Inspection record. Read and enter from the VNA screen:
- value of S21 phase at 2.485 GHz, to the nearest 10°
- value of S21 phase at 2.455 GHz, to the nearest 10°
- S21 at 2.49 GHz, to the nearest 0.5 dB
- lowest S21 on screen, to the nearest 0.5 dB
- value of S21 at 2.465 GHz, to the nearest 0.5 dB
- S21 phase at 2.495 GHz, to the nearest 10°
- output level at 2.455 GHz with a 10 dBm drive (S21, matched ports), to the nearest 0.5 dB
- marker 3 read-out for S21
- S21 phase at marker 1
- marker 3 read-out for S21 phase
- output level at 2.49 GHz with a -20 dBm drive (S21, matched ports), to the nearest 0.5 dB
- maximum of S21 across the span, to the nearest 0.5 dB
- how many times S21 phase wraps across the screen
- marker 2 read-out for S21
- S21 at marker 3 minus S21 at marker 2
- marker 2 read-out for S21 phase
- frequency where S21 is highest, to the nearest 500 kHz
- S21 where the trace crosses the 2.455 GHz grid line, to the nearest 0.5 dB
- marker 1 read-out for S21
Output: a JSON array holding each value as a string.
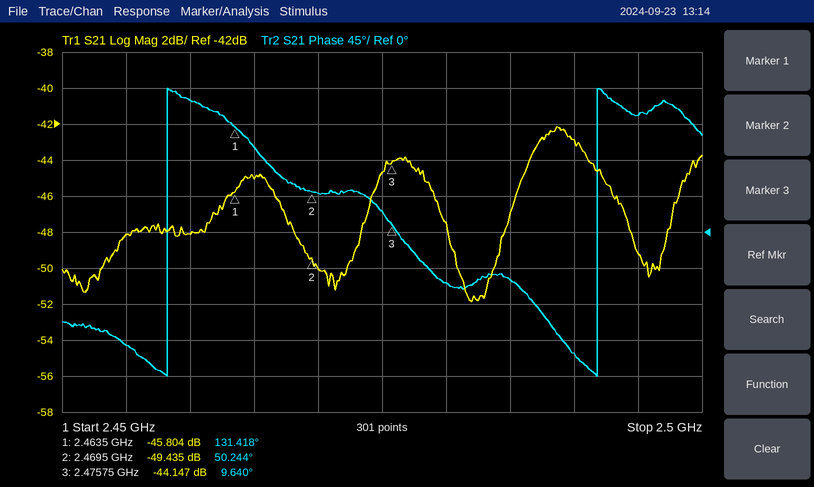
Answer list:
["-60°", "-140°", "-43.0 dB", "-52.0 dB", "-45.0 dB", "150°", "-38.0 dBm", "-44.147 dB", "131.418°", "9.640°", "-63.0 dBm", "-42.0 dB", "2", "-49.435 dB", "5.288 dB", "50.244°", "2.4885 GHz", "-48.0 dB", "-45.804 dB"]
